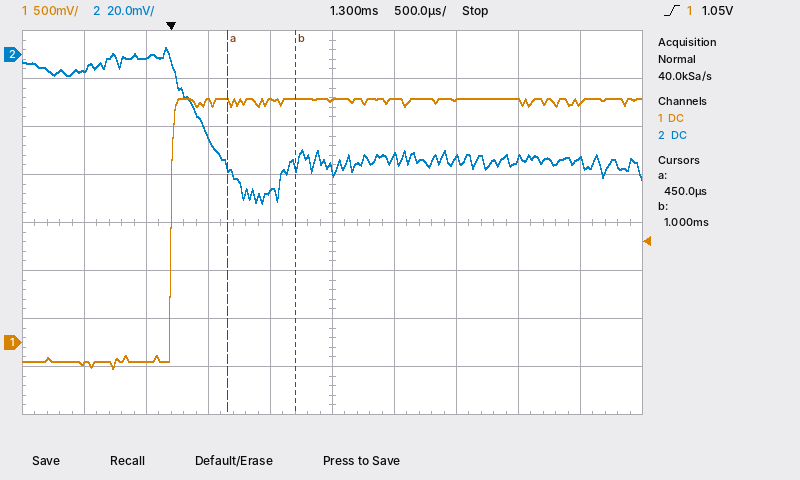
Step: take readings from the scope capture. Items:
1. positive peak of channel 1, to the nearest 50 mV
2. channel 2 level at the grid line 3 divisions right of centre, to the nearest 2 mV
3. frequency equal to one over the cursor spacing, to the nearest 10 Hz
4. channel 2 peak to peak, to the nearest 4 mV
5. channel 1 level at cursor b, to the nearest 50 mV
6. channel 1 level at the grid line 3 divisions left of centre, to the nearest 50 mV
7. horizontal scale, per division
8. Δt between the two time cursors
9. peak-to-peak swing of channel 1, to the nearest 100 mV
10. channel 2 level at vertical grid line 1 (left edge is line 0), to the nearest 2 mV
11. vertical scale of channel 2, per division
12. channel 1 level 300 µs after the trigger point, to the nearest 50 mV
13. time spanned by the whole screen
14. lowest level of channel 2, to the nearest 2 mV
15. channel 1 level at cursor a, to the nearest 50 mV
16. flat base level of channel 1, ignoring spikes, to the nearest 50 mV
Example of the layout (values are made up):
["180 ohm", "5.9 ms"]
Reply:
["2.55 V", "-44 mV", "1.82 kHz", "64 mV", "2.55 V", "-200 mV", "500 µs", "550 µs", "2.80 V", "-6 mV", "20 mV", "2.50 V", "5 ms", "-62 mV", "2.50 V", "-200 mV"]
